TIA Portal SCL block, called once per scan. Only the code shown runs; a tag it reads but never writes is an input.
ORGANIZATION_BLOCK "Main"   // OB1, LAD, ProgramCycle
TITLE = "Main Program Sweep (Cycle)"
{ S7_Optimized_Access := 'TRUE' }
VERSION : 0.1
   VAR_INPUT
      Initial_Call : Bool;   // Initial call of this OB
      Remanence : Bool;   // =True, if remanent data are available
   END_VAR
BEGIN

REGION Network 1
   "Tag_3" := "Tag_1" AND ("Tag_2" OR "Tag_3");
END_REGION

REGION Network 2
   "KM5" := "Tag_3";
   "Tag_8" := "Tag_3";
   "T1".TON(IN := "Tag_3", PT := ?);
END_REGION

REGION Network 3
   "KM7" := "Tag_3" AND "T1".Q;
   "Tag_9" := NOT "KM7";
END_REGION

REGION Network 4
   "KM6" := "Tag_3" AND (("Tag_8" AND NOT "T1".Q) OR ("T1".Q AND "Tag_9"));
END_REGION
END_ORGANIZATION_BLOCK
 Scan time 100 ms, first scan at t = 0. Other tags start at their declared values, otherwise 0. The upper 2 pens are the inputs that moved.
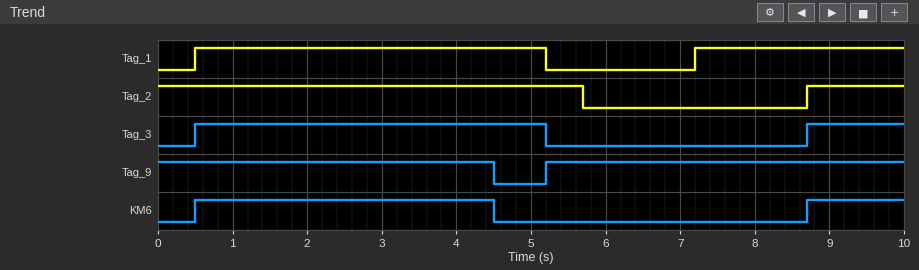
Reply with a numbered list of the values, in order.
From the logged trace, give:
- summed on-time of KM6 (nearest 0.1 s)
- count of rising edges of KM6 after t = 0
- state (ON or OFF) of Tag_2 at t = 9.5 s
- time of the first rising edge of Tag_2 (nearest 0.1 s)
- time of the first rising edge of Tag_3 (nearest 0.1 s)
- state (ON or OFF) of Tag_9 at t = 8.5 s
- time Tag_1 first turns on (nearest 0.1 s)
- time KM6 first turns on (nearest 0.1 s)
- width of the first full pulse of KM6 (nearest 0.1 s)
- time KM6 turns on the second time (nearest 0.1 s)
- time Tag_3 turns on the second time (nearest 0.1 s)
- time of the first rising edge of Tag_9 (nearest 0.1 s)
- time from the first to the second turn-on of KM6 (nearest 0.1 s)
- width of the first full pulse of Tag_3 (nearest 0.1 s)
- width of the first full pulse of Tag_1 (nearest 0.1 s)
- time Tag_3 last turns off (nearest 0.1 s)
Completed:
1. 5.3 s
2. 2
3. ON
4. 8.7 s
5. 0.5 s
6. ON
7. 0.5 s
8. 0.5 s
9. 4.0 s
10. 8.7 s
11. 8.7 s
12. 5.2 s
13. 8.2 s
14. 4.7 s
15. 4.7 s
16. 5.2 s
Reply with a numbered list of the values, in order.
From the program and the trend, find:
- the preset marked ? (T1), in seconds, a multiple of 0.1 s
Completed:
1. 4.0 s
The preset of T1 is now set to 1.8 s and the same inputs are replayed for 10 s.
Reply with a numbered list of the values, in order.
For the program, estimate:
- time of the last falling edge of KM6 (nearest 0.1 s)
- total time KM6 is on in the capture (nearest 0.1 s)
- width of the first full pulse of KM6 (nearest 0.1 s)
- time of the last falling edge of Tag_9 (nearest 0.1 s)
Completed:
1. 2.3 s
2. 3.1 s
3. 1.8 s
4. 2.3 s
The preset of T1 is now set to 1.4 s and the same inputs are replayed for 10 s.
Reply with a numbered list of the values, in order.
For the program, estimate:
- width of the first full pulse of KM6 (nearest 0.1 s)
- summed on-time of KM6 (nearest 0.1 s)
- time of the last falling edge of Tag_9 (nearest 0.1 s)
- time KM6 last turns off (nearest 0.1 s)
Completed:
1. 1.4 s
2. 2.7 s
3. 1.9 s
4. 1.9 s
